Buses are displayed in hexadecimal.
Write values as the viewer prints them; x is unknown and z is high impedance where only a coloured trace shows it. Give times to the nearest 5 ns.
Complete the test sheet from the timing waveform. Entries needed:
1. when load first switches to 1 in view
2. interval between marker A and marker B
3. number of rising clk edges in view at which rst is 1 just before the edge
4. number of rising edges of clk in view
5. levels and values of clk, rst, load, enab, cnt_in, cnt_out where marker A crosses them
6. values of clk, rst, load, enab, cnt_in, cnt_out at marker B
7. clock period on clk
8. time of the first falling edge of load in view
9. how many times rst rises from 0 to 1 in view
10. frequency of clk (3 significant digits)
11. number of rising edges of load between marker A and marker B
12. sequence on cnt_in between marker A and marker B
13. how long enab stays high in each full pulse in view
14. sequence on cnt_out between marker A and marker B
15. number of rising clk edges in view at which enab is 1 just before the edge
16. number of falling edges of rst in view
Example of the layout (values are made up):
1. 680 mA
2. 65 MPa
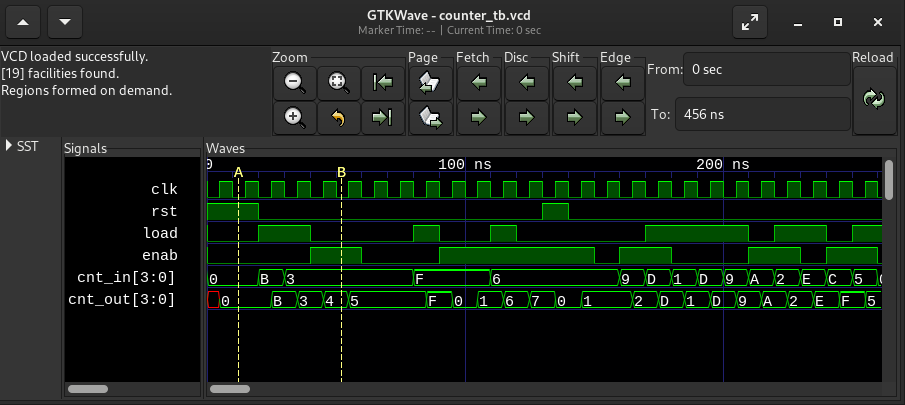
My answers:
1. 20 ns
2. 40 ns
3. 3
4. 26
5. clk=0, rst=1, load=0, enab=0, cnt_in=0, cnt_out=0
6. clk=0, rst=0, load=0, enab=1, cnt_in=3, cnt_out=4
7. 10 ns
8. 40 ns
9. 1
10. 100 MHz
11. 1
12. 0, B, 3
13. 20 ns, 60 ns, 20 ns, 20 ns, 20 ns
14. 0, B, 3, 4
15. 14
16. 2
